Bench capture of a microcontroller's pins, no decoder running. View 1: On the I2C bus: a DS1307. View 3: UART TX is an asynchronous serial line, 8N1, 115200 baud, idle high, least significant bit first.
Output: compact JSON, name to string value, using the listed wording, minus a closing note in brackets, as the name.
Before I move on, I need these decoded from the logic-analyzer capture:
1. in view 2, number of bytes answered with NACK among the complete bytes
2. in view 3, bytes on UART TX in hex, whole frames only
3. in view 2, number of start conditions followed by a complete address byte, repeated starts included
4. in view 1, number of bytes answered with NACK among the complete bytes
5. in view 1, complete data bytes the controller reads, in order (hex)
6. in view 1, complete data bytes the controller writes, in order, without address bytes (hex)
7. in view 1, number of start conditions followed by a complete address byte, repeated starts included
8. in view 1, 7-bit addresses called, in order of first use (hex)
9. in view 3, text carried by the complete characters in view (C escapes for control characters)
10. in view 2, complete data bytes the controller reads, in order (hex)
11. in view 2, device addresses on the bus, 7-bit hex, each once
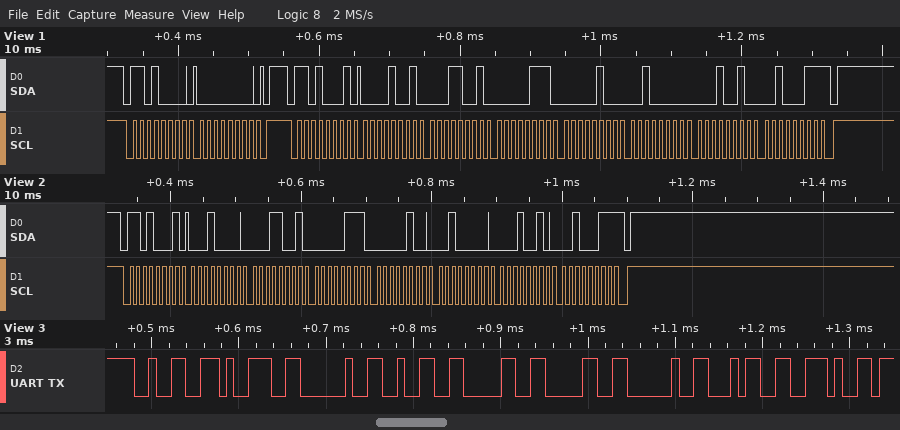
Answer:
{"in view 2, number of bytes answered with NACK among the complete bytes": "1", "in view 3, bytes on UART TX in hex, whole frames only": "0x32 0x39 0x20 0x32 0x30 0x30 0x20 0x34 0x2E", "in view 2, number of start conditions followed by a complete address byte, repeated starts included": "1", "in view 1, number of bytes answered with NACK among the complete bytes": "1", "in view 1, complete data bytes the controller reads, in order": "09 19 07 04 20 12 23", "in view 1, complete data bytes the controller writes, in order, without address bytes": "00", "in view 1, number of start conditions followed by a complete address byte, repeated starts included": "2", "in view 1, 7-bit addresses called, in order of first use": "0x68", "in view 3, text carried by the complete characters in view": "\"29 200 4.\"", "in view 2, complete data bytes the controller reads, in order": "10 19 07 04 20 12 23", "in view 2, device addresses on the bus, 7-bit hex, each once": "0x68"}
